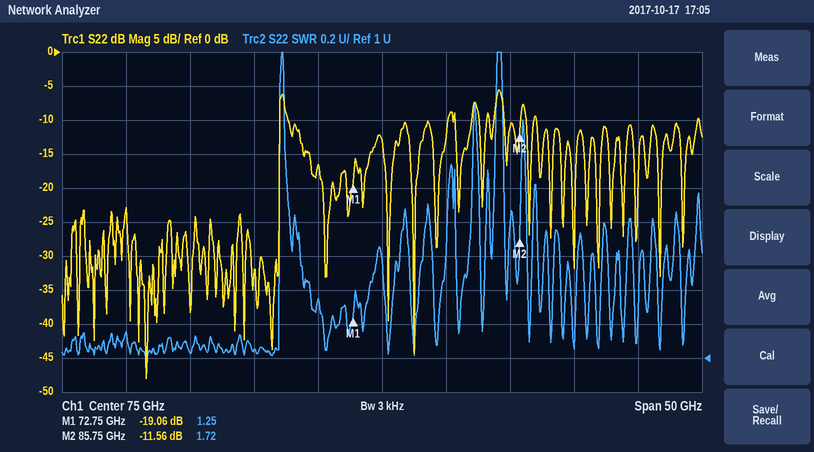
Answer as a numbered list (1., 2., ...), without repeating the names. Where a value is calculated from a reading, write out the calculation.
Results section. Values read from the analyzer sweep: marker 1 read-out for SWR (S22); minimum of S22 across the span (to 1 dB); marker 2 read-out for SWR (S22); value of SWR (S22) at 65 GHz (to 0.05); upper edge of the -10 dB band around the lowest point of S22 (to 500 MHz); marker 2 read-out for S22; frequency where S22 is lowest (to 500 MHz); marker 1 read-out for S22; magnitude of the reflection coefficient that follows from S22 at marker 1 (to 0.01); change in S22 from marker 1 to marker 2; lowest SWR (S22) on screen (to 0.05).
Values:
1. 1.25
2. -48 dB
3. 1.72
4. 1.05
5. 67.0 GHz
6. -11.56 dB
7. 56.5 GHz
8. -19.06 dB
9. 10^(-19.06/20) ≈ 0.11
10. -11.56 − (-19.06) = 7.50 dB
11. 1.00
